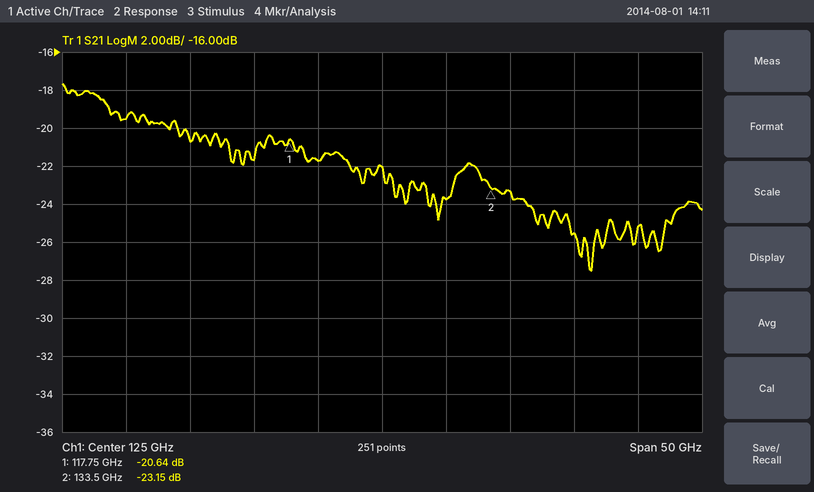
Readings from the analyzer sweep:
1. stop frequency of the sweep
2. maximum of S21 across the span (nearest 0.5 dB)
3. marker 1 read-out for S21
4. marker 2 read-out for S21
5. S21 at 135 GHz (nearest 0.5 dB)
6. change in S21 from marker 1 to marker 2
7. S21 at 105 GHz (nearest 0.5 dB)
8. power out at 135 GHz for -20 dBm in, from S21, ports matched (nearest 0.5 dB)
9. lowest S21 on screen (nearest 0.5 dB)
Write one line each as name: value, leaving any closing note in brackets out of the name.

stop frequency of the sweep: 150 GHz
maximum of S21 across the span: -17.5 dB
marker 1 read-out for S21: -20.64 dB
marker 2 read-out for S21: -23.15 dB
S21 at 135 GHz: -23.5 dB
change in S21 from marker 1 to marker 2: -2.51 dB
S21 at 105 GHz: -19.5 dB
power out at 135 GHz for -20 dBm in, from S21, ports matched: -43.5 dBm
lowest S21 on screen: -27.5 dB
